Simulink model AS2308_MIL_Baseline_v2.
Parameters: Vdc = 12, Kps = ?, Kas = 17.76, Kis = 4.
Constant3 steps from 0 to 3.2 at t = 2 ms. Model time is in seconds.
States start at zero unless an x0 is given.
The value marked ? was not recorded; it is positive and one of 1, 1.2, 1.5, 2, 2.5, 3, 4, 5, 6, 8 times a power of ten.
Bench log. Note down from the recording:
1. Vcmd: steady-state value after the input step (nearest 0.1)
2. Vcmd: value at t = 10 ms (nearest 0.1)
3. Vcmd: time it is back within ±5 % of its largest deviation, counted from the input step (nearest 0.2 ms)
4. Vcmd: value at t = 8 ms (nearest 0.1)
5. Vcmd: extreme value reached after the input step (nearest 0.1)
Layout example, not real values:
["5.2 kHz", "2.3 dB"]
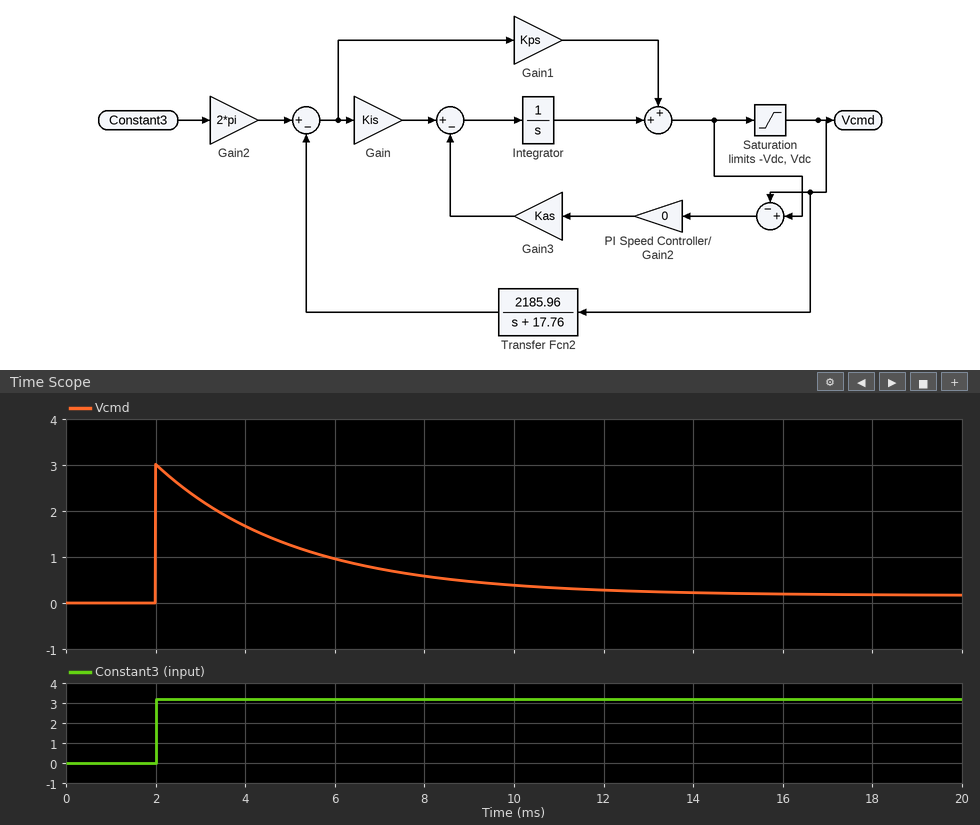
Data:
["0.2", "0.4", "9.2 ms", "0.6", "3.0"]
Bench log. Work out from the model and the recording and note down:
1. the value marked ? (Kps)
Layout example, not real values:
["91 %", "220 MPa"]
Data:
["0.15"]
